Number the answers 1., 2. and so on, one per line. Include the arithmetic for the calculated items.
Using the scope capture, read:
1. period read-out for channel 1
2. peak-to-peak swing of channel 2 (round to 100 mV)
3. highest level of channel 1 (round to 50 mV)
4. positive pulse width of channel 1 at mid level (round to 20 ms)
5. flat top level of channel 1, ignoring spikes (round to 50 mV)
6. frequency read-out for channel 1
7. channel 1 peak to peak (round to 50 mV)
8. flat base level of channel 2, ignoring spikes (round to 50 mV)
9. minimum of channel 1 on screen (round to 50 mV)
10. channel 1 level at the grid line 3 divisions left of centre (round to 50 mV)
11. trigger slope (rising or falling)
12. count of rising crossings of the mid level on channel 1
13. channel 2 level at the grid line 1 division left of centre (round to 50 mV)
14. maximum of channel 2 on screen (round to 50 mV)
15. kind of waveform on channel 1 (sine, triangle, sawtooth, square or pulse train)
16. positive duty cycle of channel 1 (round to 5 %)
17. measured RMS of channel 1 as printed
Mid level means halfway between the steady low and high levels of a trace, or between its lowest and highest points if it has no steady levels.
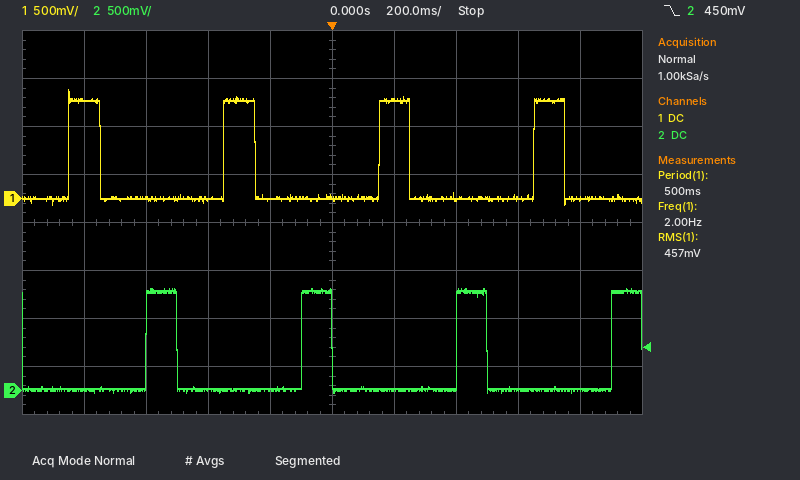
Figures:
1. 500 ms
2. 1.10 V
3. 1.15 V
4. 100 ms
5. 1.00 V
6. 2.00 Hz
7. 1.15 V − (-50 mV) = 1.20 V
8. 0 mV
9. -50 mV
10. 0 mV
11. falling
12. 4
13. 0 mV
14. 1.05 V
15. pulse train
16. 20 %
17. 457 mV
